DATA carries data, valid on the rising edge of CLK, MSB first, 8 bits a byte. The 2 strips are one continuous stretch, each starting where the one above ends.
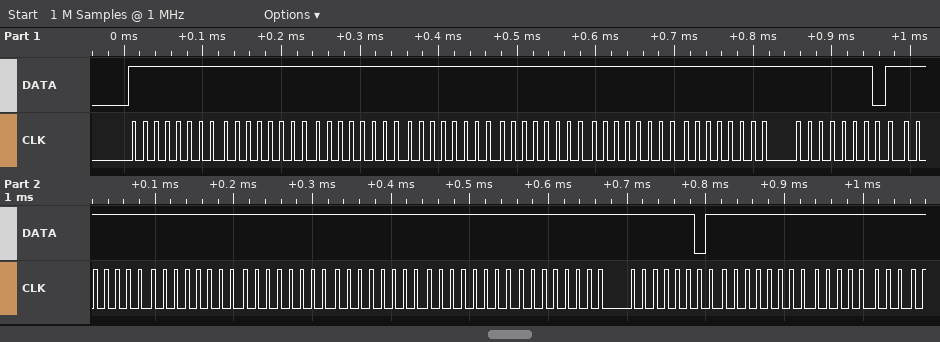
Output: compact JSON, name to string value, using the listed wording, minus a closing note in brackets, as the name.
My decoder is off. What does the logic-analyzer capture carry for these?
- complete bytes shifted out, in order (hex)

{"complete bytes shifted out, in order": "0xFF 0xFF 0xFF 0xFF 0xFF 0xFF 0xFF 0xFE 0xFF 0xFF 0xFF 0xFF 0xFF 0xFF 0xFD 0xFF 0xFF"}
